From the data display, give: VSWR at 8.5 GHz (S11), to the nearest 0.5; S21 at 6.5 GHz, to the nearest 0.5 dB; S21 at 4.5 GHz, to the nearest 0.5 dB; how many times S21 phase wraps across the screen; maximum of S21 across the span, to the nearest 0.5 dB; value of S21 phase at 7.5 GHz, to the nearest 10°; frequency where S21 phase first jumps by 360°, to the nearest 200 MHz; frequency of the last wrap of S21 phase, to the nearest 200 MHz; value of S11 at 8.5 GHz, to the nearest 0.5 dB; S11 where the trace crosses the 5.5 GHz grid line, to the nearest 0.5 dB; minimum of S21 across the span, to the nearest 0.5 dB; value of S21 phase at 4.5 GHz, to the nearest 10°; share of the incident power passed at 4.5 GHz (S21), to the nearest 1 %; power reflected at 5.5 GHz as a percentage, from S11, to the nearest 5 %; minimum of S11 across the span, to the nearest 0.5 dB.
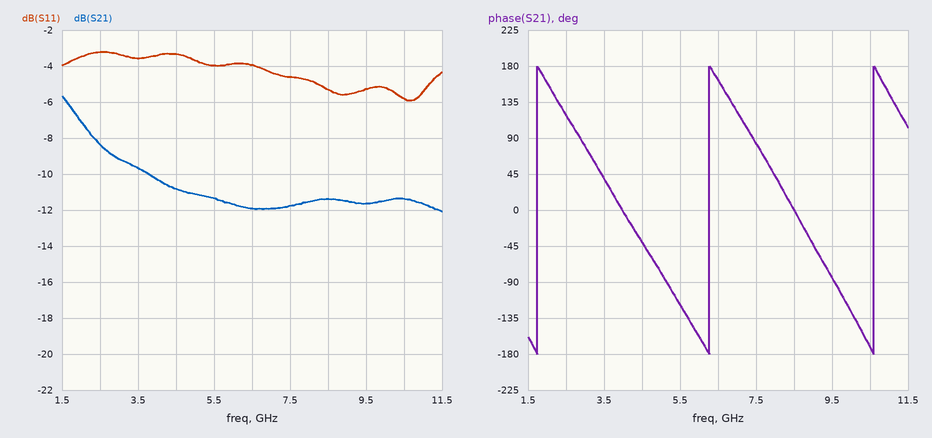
3.5
-12.0 dB
-11.0 dB
3
-5.5 dB
80°
1.8 GHz
10.6 GHz
-5.5 dB
-4.0 dB
-12.0 dB
-40°
8 %
40 %
-6.0 dB
